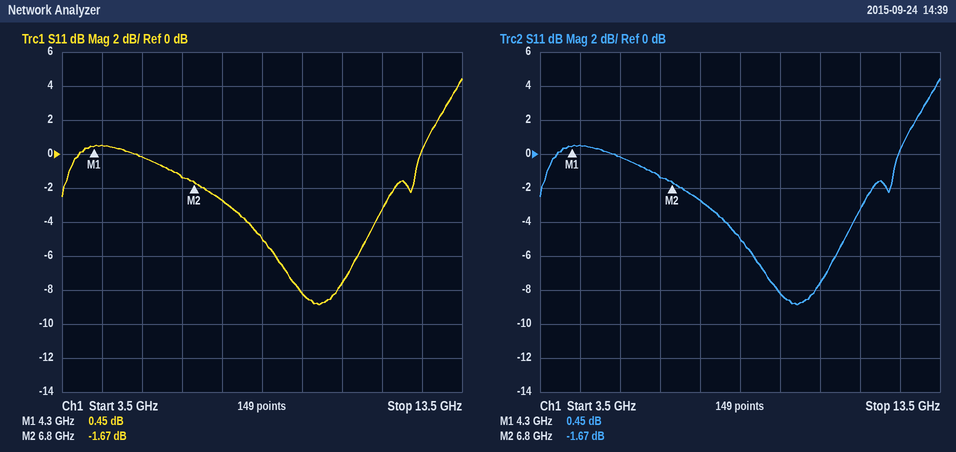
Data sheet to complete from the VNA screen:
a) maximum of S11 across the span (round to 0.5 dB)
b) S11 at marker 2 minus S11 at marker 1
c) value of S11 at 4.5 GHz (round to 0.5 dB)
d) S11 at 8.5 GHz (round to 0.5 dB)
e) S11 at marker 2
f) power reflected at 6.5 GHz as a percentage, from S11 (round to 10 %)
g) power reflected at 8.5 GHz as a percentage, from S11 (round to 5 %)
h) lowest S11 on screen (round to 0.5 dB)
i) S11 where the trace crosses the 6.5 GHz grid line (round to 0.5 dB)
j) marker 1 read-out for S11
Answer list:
4.5 dB
-2.12 dB
0.5 dB
-5.0 dB
-1.67 dB
70 %
30 %
-9.0 dB
-1.5 dB
0.45 dB
